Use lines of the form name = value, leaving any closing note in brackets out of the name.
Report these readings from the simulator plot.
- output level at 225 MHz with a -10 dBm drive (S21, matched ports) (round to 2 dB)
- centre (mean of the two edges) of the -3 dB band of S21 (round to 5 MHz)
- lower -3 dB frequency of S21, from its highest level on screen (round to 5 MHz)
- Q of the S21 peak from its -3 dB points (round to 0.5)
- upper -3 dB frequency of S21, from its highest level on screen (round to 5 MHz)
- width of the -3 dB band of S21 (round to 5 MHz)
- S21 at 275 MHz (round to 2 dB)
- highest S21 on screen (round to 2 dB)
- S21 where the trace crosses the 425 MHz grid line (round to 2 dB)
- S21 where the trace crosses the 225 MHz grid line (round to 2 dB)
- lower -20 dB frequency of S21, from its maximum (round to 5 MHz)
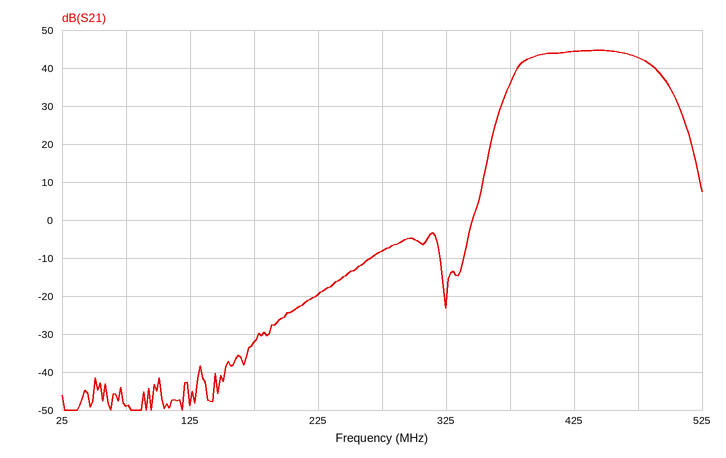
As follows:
output level at 225 MHz with a -10 dBm drive (S21, matched ports) = -30 dBm
centre (mean of the two edges) of the -3 dB band of S21 = 435 MHz
lower -3 dB frequency of S21, from its highest level on screen = 385 MHz
Q of the S21 peak from its -3 dB points = 4.5
upper -3 dB frequency of S21, from its highest level on screen = 480 MHz
width of the -3 dB band of S21 = 95 MHz
S21 at 275 MHz = -8 dB
highest S21 on screen = 44 dB
S21 where the trace crosses the 425 MHz grid line = 44 dB
S21 where the trace crosses the 225 MHz grid line = -20 dB
lower -20 dB frequency of S21, from its maximum = 365 MHz
